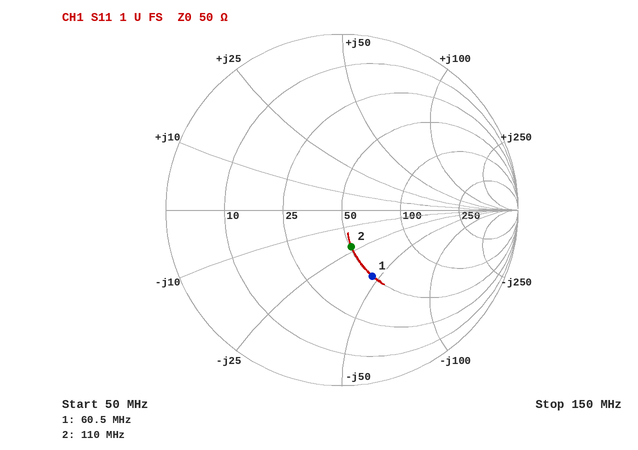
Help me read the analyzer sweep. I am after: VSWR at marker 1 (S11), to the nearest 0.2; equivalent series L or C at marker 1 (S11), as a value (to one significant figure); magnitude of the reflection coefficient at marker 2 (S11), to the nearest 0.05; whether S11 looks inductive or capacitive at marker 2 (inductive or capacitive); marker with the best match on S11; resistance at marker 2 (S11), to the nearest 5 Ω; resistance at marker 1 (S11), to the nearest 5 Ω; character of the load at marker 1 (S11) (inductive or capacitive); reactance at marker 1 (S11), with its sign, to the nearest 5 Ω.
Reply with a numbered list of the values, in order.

1. 2.4
2. 60 pF
3. 0.20
4. capacitive
5. marker 2
6. 50 Ω
7. 50 Ω
8. capacitive
9. -45 Ω
